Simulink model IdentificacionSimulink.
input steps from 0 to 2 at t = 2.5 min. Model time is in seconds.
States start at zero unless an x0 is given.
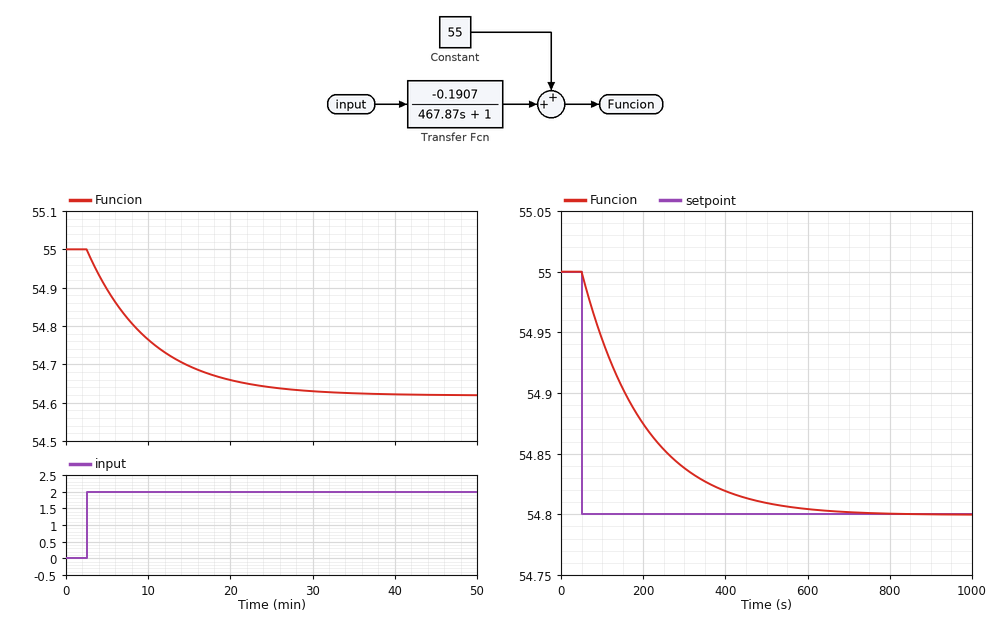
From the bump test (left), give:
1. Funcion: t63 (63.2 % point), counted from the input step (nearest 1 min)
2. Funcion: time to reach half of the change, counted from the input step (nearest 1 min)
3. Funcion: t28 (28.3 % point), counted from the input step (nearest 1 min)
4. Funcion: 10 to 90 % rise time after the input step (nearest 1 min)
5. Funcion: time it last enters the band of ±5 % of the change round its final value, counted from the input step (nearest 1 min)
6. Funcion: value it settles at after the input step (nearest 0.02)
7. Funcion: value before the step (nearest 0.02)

8 min
5 min
3 min
17 min
23 min
54.62
55.00
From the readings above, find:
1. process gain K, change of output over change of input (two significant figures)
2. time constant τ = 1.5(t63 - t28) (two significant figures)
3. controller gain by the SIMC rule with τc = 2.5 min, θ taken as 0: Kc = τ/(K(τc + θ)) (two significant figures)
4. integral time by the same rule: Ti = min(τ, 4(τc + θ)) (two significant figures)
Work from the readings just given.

-0.19
7.5 min
-16
7.5 min
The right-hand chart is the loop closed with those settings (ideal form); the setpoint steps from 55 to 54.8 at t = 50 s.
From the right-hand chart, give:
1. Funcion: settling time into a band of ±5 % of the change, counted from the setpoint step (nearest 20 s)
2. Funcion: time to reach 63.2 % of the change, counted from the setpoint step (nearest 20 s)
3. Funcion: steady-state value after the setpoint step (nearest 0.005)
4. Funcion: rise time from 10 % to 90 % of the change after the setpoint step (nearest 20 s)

440 s
160 s
54.800
320 s
